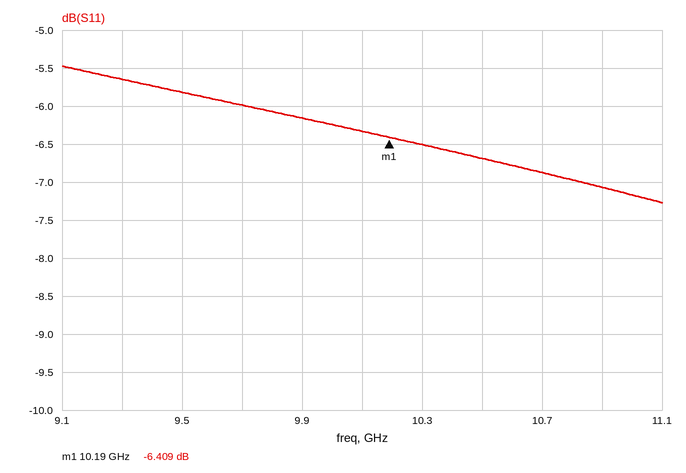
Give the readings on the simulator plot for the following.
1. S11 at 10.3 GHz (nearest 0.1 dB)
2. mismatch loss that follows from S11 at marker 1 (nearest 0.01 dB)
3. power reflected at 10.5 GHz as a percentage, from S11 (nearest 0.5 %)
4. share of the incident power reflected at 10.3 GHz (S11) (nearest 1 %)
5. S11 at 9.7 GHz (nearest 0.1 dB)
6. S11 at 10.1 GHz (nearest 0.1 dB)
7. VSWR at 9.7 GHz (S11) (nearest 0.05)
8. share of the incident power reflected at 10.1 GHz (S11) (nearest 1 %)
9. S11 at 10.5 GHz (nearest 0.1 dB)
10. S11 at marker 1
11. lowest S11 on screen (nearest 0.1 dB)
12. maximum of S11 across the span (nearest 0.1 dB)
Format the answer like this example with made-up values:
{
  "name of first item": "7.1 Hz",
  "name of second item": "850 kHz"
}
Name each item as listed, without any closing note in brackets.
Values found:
{
  "S11 at 10.3 GHz": "-6.5 dB",
  "mismatch loss that follows from S11 at marker 1": "1.13 dB",
  "power reflected at 10.5 GHz as a percentage, from S11": "21.5 %",
  "share of the incident power reflected at 10.3 GHz (S11)": "22 %",
  "S11 at 9.7 GHz": "-6.0 dB",
  "S11 at 10.1 GHz": "-6.3 dB",
  "VSWR at 9.7 GHz (S11)": "3.00",
  "share of the incident power reflected at 10.1 GHz (S11)": "23 %",
  "S11 at 10.5 GHz": "-6.7 dB",
  "S11 at marker 1": "-6.409 dB",
  "lowest S11 on screen": "-7.3 dB",
  "maximum of S11 across the span": "-5.5 dB"
}
